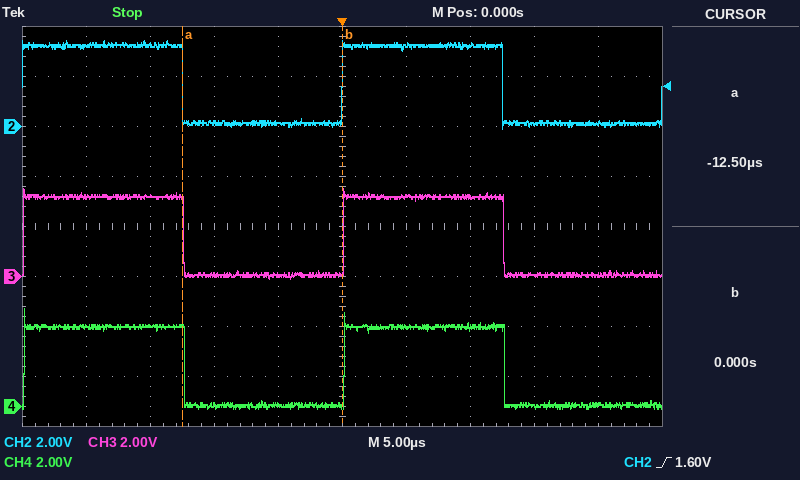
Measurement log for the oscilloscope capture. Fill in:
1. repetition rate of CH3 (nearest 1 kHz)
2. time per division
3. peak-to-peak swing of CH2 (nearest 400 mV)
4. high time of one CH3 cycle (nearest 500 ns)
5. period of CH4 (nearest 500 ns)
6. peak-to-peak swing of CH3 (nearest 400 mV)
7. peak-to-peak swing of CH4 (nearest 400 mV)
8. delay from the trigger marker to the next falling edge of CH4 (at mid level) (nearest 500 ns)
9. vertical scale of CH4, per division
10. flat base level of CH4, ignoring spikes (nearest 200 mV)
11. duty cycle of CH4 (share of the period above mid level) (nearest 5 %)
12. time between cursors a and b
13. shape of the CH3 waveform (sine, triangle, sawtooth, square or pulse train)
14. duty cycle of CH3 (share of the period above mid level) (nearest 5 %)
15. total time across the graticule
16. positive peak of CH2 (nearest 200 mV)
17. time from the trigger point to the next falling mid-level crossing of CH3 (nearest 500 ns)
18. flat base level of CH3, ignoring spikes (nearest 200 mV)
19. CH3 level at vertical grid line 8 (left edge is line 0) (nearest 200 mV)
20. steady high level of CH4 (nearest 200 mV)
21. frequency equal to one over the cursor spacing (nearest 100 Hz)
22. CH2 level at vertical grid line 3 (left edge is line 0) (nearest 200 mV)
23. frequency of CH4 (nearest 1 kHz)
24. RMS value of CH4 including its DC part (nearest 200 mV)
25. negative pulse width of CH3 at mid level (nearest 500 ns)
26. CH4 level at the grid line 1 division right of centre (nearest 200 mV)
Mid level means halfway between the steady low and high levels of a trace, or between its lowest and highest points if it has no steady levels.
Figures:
40 kHz
5 µs
3.6 V
12.5 µs
25.0 µs
3.6 V
4.0 V
12.5 µs
2 V
0.0 V
50 %
12.5 µs
square
50 %
50 µs
3.4 V
12.5 µs
0.0 V
0.0 V
3.2 V
80.0 kHz
200 mV
40 kHz
2.2 V
12.5 µs
3.2 V
